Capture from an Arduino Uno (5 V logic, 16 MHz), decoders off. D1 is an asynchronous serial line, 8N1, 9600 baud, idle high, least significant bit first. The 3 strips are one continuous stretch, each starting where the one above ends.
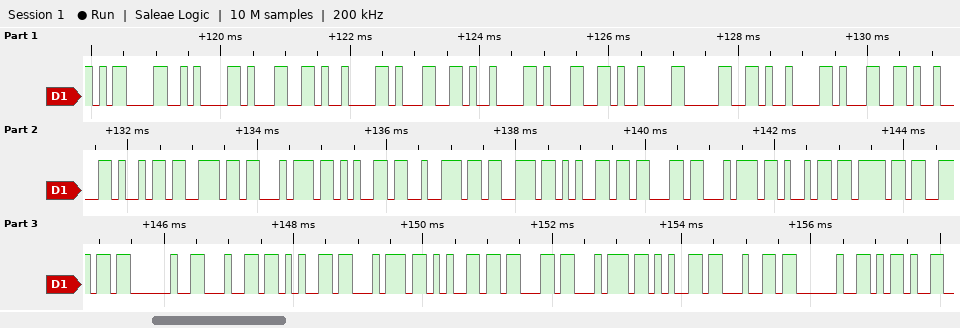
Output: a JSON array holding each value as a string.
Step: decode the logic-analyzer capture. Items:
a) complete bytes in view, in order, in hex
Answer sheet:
["0D 0A 31 09 31 09 31 09 30 09 31 09 69 6E 74 65 72 73 65 63 74 69 6F 6E 20 64 65 74 65 63 74 65 64 20 2D"]
